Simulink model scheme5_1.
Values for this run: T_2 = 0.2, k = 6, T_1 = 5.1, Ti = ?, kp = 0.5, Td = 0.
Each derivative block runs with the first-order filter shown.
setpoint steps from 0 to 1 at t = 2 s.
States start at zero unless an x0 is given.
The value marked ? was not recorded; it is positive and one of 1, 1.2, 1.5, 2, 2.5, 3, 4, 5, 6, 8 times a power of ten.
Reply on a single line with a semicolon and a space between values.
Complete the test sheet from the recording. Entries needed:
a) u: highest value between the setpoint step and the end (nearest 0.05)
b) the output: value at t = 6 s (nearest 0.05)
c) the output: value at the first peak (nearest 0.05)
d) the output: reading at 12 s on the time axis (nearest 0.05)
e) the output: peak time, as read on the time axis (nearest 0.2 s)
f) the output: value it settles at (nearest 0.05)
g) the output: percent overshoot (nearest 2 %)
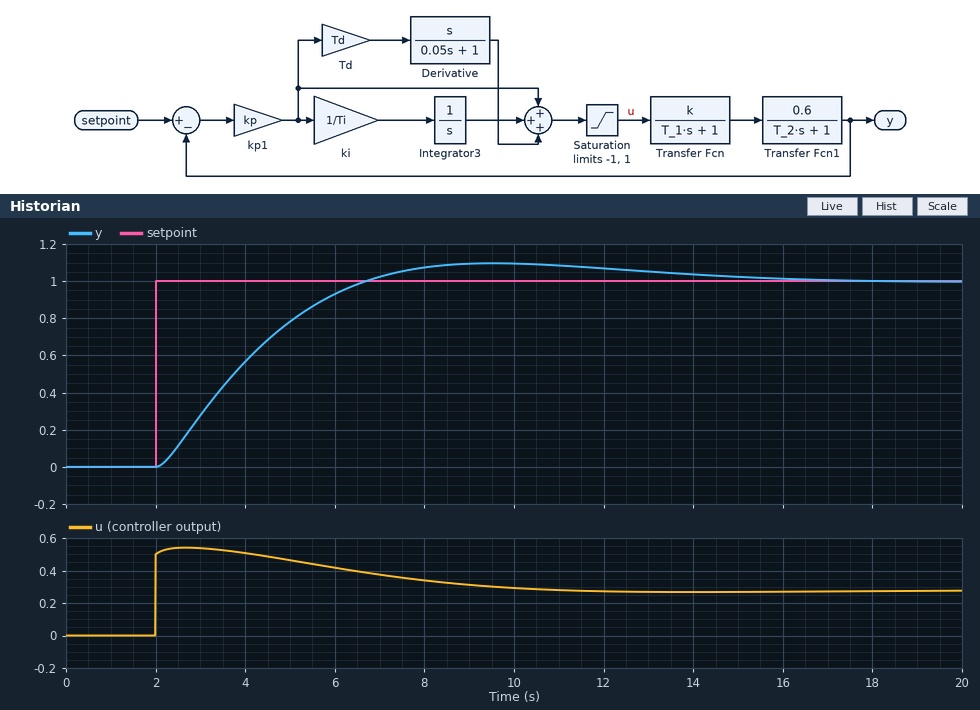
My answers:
0.55; 0.95; 1.10; 1.05; 9.6 s; 1.00; 10 %
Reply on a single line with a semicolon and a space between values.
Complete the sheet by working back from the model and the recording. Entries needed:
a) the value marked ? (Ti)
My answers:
2.5
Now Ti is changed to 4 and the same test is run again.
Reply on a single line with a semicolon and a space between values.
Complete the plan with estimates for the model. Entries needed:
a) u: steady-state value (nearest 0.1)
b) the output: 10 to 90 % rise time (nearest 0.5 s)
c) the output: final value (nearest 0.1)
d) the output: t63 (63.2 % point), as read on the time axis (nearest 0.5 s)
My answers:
0.3; 4.5 s; 1.0; 4.5 s
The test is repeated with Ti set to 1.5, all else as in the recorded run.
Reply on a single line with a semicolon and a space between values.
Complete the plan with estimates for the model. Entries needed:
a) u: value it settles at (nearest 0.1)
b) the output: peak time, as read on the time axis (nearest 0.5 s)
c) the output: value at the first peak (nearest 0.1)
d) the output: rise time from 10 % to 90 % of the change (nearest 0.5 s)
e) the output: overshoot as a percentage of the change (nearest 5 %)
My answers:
0.3; 7.5 s; 1.2; 2.5 s; 20 %
